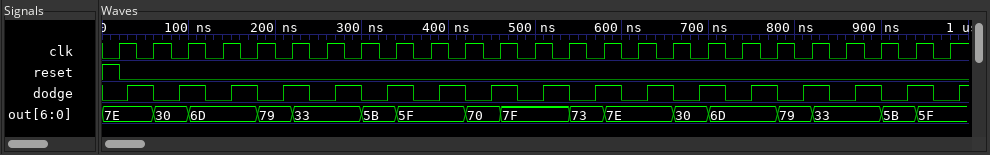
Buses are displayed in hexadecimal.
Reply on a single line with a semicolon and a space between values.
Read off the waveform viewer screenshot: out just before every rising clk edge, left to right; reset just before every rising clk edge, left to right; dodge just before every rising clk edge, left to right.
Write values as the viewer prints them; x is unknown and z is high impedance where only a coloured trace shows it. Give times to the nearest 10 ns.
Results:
7E, 7E, 30, 6D, 6D, 79, 33, 33, 5B, 5F, 5F, 70, 7F, 7F, 73, 7E, 7E, 30, 6D, 6D, 79, 33, 33, 5B, 5F; 1 0 0 0 0 0 0 0 0 0 0 0 0 0 0 0 0 0 0 0 0 0 0 0 0; 0 1 1 0 1 1 0 1 1 0 1 1 0 1 1 0 1 1 0 1 1 0 1 1 0
